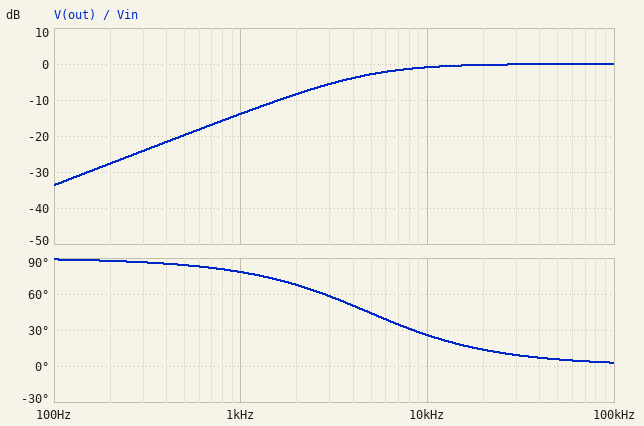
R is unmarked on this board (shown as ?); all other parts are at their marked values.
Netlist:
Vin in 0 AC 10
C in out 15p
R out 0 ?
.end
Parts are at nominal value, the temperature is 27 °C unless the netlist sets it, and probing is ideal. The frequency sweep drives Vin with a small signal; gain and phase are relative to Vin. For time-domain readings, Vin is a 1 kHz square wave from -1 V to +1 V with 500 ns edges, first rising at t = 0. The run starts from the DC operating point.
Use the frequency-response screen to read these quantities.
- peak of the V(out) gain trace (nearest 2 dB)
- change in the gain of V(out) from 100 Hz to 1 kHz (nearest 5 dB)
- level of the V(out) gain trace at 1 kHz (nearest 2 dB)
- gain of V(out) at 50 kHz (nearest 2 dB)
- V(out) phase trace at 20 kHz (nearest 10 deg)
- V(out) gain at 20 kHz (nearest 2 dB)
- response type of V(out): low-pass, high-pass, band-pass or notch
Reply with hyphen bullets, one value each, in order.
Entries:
- 0 dB
- 20 dB
- -14 dB
- 0 dB
- 10 deg
- 0 dB
- high-pass
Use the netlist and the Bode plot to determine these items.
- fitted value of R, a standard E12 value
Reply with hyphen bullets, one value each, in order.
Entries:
- 2.2 MΩ
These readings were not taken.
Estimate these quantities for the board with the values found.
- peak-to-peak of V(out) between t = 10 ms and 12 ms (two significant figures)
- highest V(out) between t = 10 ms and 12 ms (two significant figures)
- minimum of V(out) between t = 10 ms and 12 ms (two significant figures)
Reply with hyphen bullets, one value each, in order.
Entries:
- 4.0 V
- 2.0 V
- -2.0 V
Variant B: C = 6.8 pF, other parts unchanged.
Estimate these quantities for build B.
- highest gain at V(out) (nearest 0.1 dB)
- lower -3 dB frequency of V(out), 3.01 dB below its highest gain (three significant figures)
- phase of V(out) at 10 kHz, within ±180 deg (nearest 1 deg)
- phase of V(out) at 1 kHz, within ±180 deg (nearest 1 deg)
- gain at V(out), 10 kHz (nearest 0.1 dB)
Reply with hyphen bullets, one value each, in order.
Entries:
- 0 dB
- 10.6 kHz
- 47 deg
- 85 deg
- -3.3 dB
